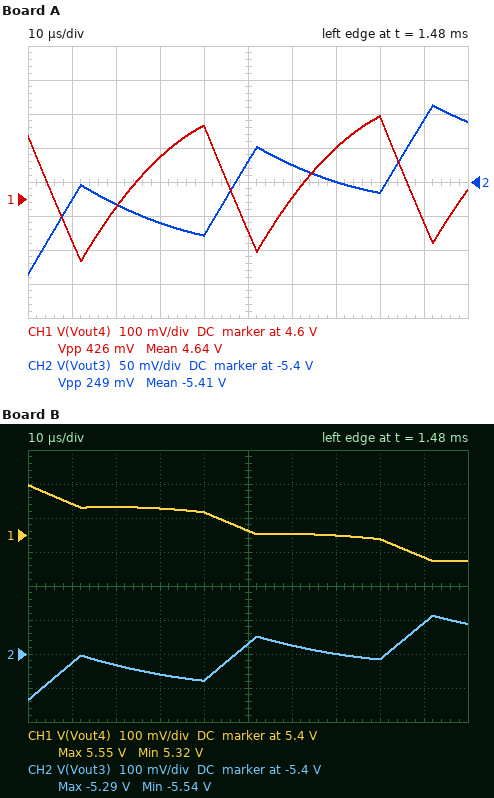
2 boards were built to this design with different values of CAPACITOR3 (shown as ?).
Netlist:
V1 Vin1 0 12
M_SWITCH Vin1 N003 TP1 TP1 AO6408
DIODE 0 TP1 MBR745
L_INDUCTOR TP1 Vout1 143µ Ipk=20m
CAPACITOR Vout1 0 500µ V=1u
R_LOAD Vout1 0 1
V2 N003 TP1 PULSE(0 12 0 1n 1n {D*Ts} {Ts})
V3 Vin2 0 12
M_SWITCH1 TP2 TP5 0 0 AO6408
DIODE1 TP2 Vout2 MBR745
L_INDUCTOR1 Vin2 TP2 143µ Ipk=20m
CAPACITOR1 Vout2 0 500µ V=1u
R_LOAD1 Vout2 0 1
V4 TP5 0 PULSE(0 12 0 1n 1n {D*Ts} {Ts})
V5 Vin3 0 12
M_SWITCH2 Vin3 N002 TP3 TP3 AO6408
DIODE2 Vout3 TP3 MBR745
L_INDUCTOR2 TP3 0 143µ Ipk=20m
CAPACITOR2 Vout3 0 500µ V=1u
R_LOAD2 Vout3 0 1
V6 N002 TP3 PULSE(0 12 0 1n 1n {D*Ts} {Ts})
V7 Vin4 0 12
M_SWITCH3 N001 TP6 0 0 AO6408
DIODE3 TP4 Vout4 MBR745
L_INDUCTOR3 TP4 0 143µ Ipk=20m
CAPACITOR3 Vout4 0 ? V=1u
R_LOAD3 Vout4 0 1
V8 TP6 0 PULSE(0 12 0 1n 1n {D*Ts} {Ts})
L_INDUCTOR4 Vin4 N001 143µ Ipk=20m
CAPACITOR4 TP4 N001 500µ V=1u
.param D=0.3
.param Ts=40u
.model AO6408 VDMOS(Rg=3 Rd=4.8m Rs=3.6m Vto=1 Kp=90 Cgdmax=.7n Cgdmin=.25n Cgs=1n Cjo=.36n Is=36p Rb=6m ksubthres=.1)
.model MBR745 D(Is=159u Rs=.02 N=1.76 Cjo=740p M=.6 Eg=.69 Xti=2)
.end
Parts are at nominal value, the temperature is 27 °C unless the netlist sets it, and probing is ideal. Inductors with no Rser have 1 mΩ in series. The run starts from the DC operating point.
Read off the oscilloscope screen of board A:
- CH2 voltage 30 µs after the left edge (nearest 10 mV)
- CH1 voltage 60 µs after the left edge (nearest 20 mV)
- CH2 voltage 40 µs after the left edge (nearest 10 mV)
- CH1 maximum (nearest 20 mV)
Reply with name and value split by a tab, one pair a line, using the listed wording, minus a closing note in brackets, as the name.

CH2 voltage 30 µs after the left edge	-5.46 V
CH1 voltage 60 µs after the left edge	4.60 V
CH2 voltage 40 µs after the left edge	-5.48 V
CH1 maximum	4.84 V
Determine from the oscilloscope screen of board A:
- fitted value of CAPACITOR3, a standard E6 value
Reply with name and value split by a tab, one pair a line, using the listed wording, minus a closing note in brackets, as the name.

fitted value of CAPACITOR3, a standard E6 value	150 µF
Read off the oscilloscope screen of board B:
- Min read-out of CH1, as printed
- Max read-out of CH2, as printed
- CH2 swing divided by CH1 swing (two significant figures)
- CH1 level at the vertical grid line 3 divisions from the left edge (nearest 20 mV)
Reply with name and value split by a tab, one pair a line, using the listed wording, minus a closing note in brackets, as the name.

Min read-out of CH1, as printed	5.32 V
Max read-out of CH2, as printed	-5.29 V
CH2 swing divided by CH1 swing	1.1
CH1 level at the vertical grid line 3 divisions from the left edge	5.48 V
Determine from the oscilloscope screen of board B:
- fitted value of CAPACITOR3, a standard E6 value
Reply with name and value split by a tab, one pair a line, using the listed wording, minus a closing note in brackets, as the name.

fitted value of CAPACITOR3, a standard E6 value	1 mF
